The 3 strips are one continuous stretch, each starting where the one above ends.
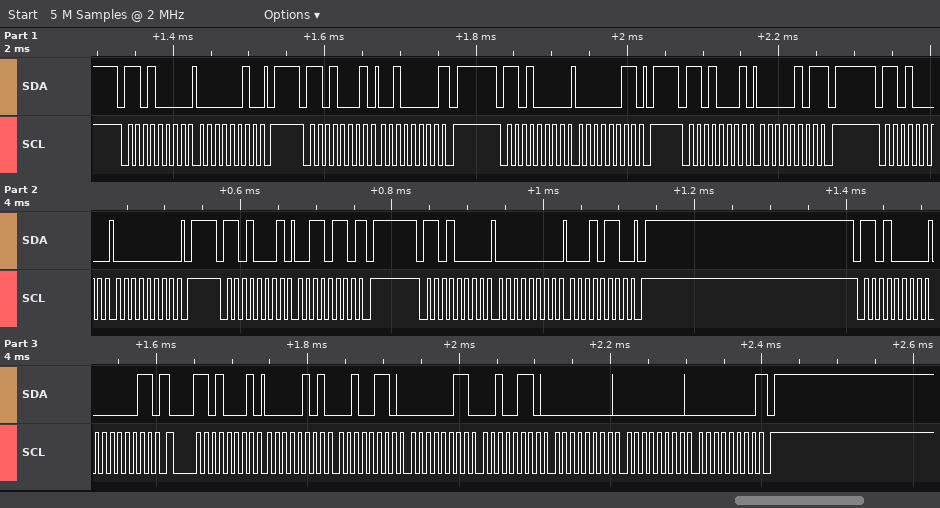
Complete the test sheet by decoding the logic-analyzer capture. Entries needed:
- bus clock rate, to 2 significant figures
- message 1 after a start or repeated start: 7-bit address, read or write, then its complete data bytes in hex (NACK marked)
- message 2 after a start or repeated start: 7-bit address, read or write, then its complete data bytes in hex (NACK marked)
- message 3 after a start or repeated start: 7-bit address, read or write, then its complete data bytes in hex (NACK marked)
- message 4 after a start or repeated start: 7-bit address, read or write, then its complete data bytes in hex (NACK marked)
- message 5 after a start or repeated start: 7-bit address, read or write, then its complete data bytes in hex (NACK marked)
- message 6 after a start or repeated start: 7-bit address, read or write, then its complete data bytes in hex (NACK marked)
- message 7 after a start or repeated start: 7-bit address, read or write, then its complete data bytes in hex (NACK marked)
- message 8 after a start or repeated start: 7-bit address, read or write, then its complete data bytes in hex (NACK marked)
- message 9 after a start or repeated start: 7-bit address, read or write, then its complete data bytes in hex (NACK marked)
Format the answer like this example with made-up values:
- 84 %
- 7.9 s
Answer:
- 100 kHz
- 0x68 write: 02
- 0x68 read: 20 NACK
- 0x68 write: 03
- 0x68 read: 05 NACK
- 0x68 write: 00
- 0x68 read: 36 NACK
- 0x68 write: 00 16
- 0x68 write: 03
- 0x68 read: 05 26 03 26 00 00 00 NACK
